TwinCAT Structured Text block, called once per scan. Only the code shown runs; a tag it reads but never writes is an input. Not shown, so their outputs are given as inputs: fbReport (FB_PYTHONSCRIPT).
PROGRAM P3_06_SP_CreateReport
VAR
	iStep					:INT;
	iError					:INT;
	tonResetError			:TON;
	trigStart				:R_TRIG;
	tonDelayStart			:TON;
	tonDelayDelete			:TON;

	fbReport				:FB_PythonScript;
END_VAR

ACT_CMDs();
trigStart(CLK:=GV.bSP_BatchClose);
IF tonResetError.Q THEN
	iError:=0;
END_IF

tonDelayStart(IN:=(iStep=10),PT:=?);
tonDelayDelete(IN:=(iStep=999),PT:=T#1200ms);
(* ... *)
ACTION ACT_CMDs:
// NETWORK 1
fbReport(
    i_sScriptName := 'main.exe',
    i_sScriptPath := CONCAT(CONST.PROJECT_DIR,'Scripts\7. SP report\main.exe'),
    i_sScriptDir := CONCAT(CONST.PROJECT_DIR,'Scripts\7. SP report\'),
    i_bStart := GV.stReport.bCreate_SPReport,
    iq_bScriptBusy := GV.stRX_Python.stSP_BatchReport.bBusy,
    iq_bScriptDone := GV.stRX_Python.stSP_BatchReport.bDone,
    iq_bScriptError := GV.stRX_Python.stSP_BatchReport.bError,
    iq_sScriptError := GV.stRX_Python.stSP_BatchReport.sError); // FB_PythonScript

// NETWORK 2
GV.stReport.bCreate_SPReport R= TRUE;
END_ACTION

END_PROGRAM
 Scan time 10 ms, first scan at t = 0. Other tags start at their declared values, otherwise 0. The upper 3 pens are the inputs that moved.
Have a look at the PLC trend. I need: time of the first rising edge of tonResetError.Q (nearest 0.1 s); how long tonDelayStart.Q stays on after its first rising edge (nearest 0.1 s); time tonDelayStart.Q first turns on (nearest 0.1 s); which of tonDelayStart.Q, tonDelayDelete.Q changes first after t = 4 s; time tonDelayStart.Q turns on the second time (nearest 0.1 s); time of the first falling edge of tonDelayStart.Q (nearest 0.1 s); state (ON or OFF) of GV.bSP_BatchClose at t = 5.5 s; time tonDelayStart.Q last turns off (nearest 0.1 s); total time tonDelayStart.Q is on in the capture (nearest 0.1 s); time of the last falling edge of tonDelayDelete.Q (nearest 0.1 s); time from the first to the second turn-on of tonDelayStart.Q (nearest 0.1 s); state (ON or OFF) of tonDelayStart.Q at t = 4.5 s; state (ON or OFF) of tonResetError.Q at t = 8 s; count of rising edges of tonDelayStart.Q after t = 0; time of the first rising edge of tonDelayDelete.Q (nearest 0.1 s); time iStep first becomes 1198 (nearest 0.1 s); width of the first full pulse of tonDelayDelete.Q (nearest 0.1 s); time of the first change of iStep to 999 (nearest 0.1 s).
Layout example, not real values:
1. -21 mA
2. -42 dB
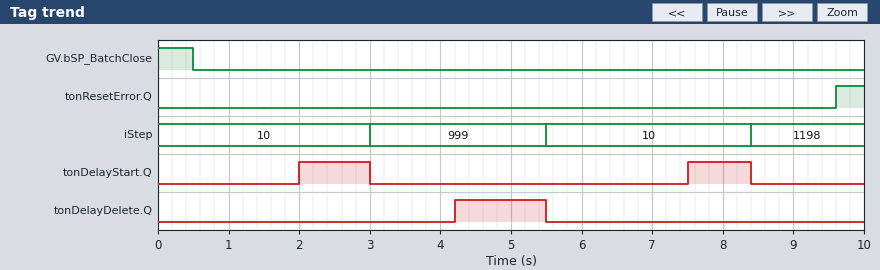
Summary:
1. 9.6 s
2. 1.0 s
3. 2.0 s
4. tonDelayDelete.Q
5. 7.5 s
6. 3.0 s
7. OFF
8. 8.4 s
9. 1.9 s
10. 5.5 s
11. 5.5 s
12. OFF
13. OFF
14. 2
15. 4.2 s
16. 8.4 s
17. 1.3 s
18. 3.0 s
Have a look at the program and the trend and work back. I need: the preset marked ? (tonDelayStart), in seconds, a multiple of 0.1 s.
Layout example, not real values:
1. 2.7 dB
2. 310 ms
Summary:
1. 2.0 s
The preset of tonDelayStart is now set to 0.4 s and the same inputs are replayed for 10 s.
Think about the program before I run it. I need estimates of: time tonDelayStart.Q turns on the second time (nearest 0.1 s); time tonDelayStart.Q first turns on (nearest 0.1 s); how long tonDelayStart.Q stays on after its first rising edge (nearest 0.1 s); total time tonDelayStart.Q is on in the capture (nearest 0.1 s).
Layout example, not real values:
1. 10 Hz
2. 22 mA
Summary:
1. 5.9 s
2. 0.4 s
3. 2.6 s
4. 5.1 s
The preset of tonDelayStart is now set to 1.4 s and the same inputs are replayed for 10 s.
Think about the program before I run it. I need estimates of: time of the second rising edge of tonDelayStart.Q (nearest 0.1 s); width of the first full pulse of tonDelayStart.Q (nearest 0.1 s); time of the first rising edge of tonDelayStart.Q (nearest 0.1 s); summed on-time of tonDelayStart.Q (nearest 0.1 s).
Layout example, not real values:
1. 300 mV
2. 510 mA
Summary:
1. 6.9 s
2. 1.6 s
3. 1.4 s
4. 3.1 s
